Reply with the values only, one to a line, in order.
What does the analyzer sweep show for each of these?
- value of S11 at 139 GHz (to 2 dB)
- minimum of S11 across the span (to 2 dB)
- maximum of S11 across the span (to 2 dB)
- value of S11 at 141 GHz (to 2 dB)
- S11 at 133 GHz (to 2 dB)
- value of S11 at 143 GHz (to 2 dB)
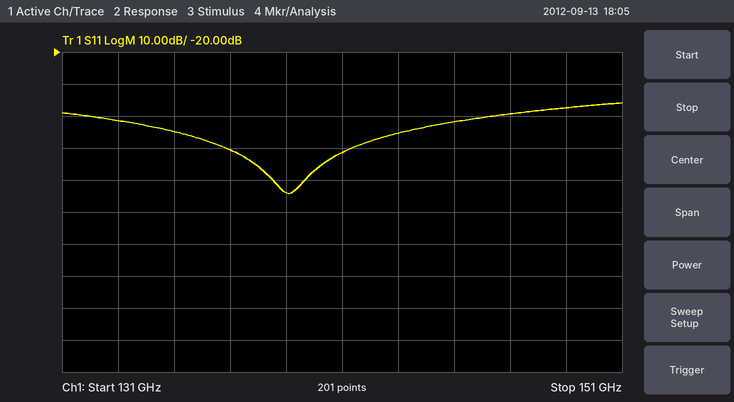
-64 dB
-64 dB
-36 dB
-52 dB
-42 dB
-46 dB
